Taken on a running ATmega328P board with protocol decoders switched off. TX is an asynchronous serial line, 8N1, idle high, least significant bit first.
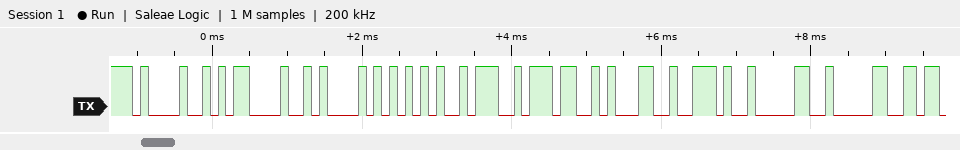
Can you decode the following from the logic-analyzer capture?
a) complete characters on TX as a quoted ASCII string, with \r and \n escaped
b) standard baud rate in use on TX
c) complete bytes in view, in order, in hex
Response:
"!\r\nU:71.00"
9600 baud
21 0D 0A 55 3A 37 31 2E 30 30
